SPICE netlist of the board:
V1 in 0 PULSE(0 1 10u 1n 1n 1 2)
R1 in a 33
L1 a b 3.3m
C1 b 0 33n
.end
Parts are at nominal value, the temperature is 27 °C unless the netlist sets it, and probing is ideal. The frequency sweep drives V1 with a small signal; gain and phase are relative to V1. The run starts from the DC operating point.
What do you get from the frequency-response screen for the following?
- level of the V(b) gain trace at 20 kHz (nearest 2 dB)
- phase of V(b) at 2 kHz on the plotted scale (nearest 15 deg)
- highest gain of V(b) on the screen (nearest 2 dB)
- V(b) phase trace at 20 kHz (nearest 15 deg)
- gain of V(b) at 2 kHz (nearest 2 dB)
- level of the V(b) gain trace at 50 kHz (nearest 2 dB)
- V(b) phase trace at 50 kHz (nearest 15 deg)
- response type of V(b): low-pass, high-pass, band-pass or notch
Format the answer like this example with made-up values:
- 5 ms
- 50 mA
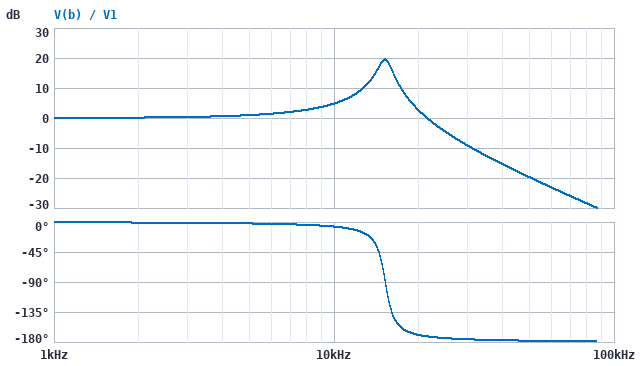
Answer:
- 2 dB
- 0 deg
- 20 dB
- -165 deg
- 0 dB
- -20 dB
- -180 deg
- low-pass
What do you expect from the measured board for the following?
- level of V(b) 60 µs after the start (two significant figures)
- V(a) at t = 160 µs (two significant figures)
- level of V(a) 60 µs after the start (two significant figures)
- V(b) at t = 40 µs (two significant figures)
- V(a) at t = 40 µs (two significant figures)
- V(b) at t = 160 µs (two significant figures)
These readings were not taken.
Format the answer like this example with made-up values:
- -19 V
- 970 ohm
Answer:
- 980 mV
- 950 mV
- 1.1 V
- 1.8 V
- 980 mV
- 1.1 V
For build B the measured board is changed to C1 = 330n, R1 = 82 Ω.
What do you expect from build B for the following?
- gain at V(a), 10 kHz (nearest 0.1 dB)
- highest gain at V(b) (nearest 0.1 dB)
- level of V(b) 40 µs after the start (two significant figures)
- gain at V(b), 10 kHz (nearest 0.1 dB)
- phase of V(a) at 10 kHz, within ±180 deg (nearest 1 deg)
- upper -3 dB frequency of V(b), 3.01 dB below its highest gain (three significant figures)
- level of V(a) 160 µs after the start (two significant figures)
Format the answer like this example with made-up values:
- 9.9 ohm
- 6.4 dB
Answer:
- -1.0 dB
- 2.5 dB
- 310 mV
- -11.4 dB
- 27 deg
- 5.73 kHz
- 1.1 V
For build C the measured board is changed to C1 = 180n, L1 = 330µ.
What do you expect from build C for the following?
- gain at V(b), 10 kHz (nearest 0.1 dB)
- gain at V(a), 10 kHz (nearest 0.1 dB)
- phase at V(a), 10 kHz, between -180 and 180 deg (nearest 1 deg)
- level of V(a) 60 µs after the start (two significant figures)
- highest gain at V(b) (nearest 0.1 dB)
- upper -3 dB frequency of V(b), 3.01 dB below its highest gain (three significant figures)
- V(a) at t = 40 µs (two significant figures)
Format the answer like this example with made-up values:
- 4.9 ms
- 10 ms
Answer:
- 1.4 dB
- -0.9 dB
- -26 deg
- 1.0 V
- 3.0 dB
- 24.6 kHz
- 1.1 V
